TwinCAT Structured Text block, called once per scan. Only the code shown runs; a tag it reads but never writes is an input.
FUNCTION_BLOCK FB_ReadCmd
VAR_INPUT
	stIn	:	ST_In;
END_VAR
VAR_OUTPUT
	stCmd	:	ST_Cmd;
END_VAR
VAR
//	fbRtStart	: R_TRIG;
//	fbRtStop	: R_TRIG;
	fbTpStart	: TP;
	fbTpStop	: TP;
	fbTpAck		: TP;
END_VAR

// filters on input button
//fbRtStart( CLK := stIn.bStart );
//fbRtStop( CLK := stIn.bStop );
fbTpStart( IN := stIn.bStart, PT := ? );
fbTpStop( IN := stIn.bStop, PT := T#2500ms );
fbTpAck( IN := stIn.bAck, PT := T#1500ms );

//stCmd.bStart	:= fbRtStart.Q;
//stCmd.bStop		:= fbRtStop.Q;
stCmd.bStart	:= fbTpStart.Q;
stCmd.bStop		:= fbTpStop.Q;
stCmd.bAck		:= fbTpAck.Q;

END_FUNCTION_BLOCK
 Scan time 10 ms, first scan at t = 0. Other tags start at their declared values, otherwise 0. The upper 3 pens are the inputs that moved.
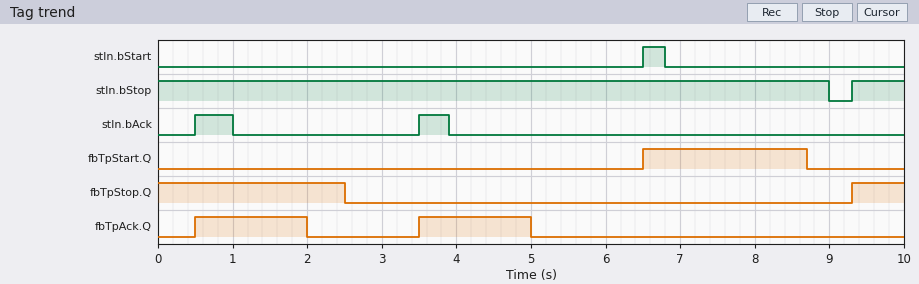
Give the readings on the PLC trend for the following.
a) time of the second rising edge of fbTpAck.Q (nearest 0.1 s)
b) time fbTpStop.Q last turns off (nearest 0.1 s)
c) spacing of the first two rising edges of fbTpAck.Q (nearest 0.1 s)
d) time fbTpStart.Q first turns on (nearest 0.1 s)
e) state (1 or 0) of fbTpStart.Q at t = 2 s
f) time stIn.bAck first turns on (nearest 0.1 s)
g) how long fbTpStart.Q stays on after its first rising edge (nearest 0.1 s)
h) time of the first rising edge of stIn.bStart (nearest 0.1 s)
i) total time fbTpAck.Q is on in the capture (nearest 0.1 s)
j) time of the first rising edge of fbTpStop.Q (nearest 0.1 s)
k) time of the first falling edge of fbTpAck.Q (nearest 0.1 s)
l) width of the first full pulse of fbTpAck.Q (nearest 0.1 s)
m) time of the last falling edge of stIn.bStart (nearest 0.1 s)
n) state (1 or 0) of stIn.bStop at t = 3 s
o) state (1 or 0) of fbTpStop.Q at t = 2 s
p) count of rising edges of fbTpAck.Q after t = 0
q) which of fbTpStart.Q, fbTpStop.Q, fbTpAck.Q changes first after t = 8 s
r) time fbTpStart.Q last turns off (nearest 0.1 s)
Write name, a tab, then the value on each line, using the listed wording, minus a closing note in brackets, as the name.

time of the second rising edge of fbTpAck.Q	3.5 s
time fbTpStop.Q last turns off	2.5 s
spacing of the first two rising edges of fbTpAck.Q	3.0 s
time fbTpStart.Q first turns on	6.5 s
state (1 or 0) of fbTpStart.Q at t = 2 s	0
time stIn.bAck first turns on	0.5 s
how long fbTpStart.Q stays on after its first rising edge	2.2 s
time of the first rising edge of stIn.bStart	6.5 s
total time fbTpAck.Q is on in the capture	3.0 s
time of the first rising edge of fbTpStop.Q	9.3 s
time of the first falling edge of fbTpAck.Q	2.0 s
width of the first full pulse of fbTpAck.Q	1.5 s
time of the last falling edge of stIn.bStart	6.8 s
state (1 or 0) of stIn.bStop at t = 3 s	1
state (1 or 0) of fbTpStop.Q at t = 2 s	1
count of rising edges of fbTpAck.Q after t = 0	2
which of fbTpStart.Q, fbTpStop.Q, fbTpAck.Q changes first after t = 8 s	fbTpStart.Q
time fbTpStart.Q last turns off	8.7 s
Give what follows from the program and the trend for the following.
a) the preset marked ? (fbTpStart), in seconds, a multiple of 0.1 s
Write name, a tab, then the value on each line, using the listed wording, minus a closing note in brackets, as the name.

the preset marked ? (fbTpStart), in seconds, a multiple of 0.1 s	2.2 s
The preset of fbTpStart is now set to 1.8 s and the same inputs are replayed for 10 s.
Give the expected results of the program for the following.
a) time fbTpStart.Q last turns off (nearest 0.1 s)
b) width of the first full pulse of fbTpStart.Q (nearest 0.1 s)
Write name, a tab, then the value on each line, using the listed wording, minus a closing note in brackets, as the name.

time fbTpStart.Q last turns off	8.3 s
width of the first full pulse of fbTpStart.Q	1.8 s
